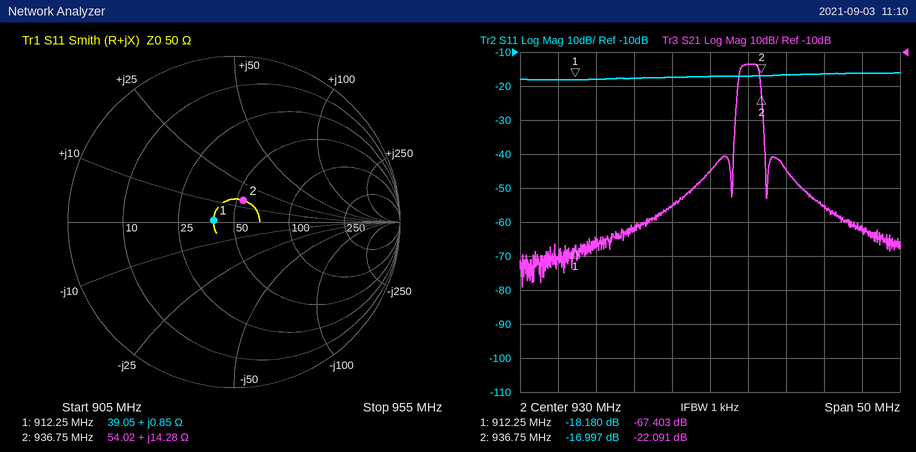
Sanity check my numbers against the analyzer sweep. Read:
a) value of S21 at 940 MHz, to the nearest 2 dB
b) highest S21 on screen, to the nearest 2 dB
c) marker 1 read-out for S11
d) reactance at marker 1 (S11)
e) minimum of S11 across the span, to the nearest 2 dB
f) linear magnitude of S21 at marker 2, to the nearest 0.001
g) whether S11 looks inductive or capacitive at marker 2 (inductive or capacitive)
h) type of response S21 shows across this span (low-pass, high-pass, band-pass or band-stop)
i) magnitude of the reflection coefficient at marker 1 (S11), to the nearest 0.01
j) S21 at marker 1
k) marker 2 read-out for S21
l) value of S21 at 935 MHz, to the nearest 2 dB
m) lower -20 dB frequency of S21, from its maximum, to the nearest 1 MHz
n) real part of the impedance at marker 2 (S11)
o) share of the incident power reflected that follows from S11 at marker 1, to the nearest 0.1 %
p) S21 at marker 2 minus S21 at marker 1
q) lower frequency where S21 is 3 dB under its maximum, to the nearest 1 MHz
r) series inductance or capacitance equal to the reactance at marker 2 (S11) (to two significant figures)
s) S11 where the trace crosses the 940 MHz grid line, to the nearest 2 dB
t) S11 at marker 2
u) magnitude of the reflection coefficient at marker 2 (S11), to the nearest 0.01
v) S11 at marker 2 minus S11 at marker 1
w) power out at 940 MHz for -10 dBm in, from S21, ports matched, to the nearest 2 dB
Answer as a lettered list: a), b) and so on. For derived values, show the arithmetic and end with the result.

a) -44 dB
b) -14 dB
c) -18.180 dB
d) +0.85 Ω
e) -18 dB
f) 10^(-22.091/20) ≈ 0.079
g) inductive
h) band-pass
i) 0.12
j) -67.403 dB
k) -22.091 dB
l) -14 dB
m) 933 MHz
n) 54.02 Ω
o) 10^(-18.18/10) ≈ 1.5 %
p) -22.091 − (-67.403) = 45.312 dB
q) 934 MHz
r) L = 14.28 Ω/(2π × 936.75 MHz) ≈ 2.4 nH
s) -16 dB
t) -16.997 dB
u) 0.14
v) -16.997 − (-18.18) = 1.183 dB
w) -10 dBm + (-44 dB) = -54 dBm
